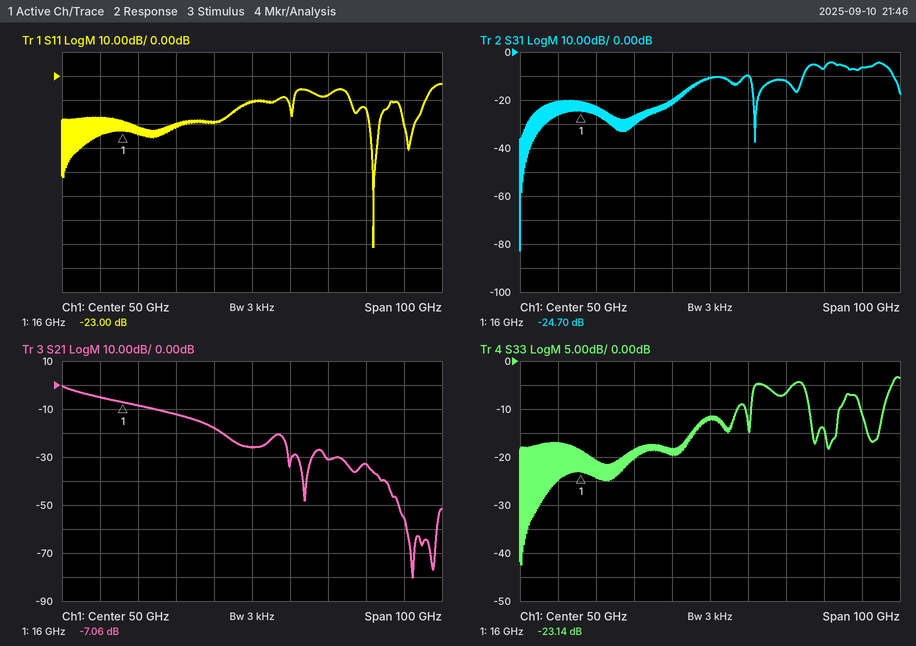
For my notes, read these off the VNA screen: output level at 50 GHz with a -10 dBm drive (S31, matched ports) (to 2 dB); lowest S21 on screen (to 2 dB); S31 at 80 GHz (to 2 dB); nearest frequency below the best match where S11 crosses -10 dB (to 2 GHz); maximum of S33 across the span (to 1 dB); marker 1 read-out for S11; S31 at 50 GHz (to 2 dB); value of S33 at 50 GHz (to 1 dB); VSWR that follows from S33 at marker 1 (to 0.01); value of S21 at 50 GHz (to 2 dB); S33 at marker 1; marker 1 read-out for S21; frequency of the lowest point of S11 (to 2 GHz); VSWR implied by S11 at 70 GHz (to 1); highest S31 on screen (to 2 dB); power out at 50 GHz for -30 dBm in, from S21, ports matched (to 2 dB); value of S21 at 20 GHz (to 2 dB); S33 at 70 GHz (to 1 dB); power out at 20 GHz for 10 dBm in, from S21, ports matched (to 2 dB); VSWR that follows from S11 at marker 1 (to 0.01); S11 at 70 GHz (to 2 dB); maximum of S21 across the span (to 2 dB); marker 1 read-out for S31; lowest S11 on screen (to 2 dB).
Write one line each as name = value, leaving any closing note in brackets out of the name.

output level at 50 GHz with a -10 dBm drive (S31, matched ports) = -20 dBm
lowest S21 on screen = -80 dB
S31 at 80 GHz = -6 dB
nearest frequency below the best match where S11 crosses -10 dB = 76 GHz
maximum of S33 across the span = -3 dB
marker 1 read-out for S11 = -23.00 dB
S31 at 50 GHz = -10 dB
value of S33 at 50 GHz = -12 dB
VSWR that follows from S33 at marker 1 = 1.15
value of S21 at 50 GHz = -26 dB
S33 at marker 1 = -23.14 dB
marker 1 read-out for S21 = -7.06 dB
frequency of the lowest point of S11 = 82 GHz
VSWR implied by S11 at 70 GHz = 2
highest S31 on screen = -4 dB
power out at 50 GHz for -30 dBm in, from S21, ports matched = -56 dBm
value of S21 at 20 GHz = -8 dB
S33 at 70 GHz = -7 dB
power out at 20 GHz for 10 dBm in, from S21, ports matched = 2 dBm
VSWR that follows from S11 at marker 1 = 1.15
S11 at 70 GHz = -8 dB
maximum of S21 across the span = 0 dB
marker 1 read-out for S31 = -24.70 dB
lowest S11 on screen = -72 dB
